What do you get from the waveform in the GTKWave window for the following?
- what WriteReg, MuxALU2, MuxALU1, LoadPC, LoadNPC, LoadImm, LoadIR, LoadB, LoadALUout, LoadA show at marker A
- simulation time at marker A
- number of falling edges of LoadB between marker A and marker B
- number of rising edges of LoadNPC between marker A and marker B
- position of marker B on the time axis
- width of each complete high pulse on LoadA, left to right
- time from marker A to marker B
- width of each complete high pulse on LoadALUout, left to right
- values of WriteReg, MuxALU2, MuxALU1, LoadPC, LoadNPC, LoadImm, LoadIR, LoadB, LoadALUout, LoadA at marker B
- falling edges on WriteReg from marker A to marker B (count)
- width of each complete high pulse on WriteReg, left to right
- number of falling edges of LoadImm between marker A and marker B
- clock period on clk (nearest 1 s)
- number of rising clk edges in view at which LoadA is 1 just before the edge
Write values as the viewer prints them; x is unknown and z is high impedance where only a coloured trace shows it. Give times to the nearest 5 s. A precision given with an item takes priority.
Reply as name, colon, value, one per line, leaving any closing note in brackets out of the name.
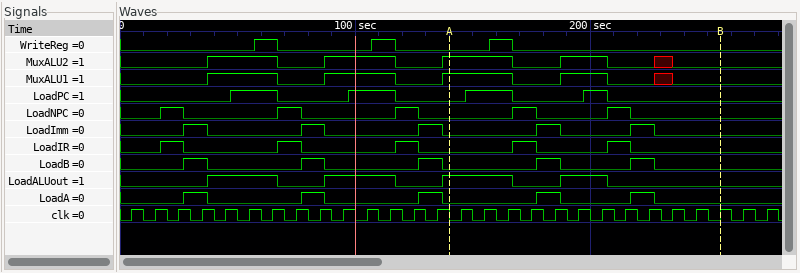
what WriteReg, MuxALU2, MuxALU1, LoadPC, LoadNPC, LoadImm, LoadIR, LoadB, LoadALUout, LoadA show at marker A: WriteReg=0, MuxALU2=1, MuxALU1=1, LoadPC=0, LoadNPC=0, LoadImm=0, LoadIR=0, LoadB=0, LoadALUout=1, LoadA=0
simulation time at marker A: 140 s
number of falling edges of LoadB between marker A and marker B: 2
number of rising edges of LoadNPC between marker A and marker B: 2
position of marker B on the time axis: 255 s
width of each complete high pulse on LoadA, left to right: 10 s, 10 s, 10 s, 10 s, 10 s
time from marker A to marker B: 115 s
width of each complete high pulse on LoadALUout, left to right: 30 s, 30 s, 30 s, 20 s
values of WriteReg, MuxALU2, MuxALU1, LoadPC, LoadNPC, LoadImm, LoadIR, LoadB, LoadALUout, LoadA at marker B: WriteReg=0, MuxALU2=0, MuxALU1=0, LoadPC=0, LoadNPC=0, LoadImm=0, LoadIR=0, LoadB=0, LoadALUout=0, LoadA=0
falling edges on WriteReg from marker A to marker B: 1
width of each complete high pulse on WriteReg, left to right: 10 s, 10 s, 10 s
number of falling edges of LoadImm between marker A and marker B: 2
clock period on clk: 10 s
number of rising clk edges in view at which LoadA is 1 just before the edge: 5
